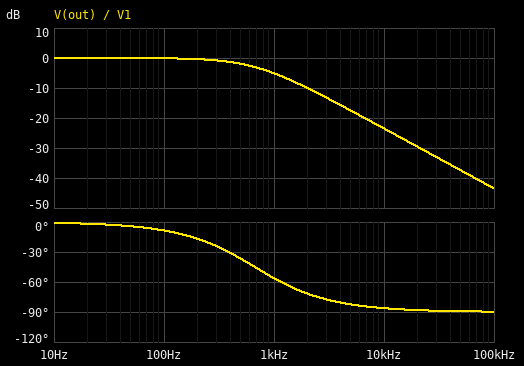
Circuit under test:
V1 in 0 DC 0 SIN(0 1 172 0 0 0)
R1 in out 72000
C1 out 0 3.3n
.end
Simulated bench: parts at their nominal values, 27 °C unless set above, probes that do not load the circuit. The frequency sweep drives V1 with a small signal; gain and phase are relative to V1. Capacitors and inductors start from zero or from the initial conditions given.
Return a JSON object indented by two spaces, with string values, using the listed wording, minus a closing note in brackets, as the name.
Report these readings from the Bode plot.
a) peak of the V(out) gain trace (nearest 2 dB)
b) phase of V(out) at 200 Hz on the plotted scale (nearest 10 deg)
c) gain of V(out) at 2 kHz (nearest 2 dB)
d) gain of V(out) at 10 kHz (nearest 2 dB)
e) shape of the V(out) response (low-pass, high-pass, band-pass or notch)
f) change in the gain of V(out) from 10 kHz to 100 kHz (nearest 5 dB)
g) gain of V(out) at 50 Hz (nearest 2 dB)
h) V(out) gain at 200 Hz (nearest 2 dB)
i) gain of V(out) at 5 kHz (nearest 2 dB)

{
  "peak of the V(out) gain trace": "0 dB",
  "phase of V(out) at 200 Hz on the plotted scale": "-20 deg",
  "gain of V(out) at 2 kHz": "-10 dB",
  "gain of V(out) at 10 kHz": "-24 dB",
  "shape of the V(out) response": "low-pass",
  "change in the gain of V(out) from 10 kHz to 100 kHz": "-20 dB",
  "gain of V(out) at 50 Hz": "0 dB",
  "V(out) gain at 200 Hz": "0 dB",
  "gain of V(out) at 5 kHz": "-18 dB"
}
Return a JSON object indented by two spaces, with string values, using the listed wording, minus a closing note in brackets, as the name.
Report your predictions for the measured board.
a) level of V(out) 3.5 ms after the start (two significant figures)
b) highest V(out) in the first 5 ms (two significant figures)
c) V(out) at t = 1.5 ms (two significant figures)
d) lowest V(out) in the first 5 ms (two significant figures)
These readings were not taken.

{
  "level of V(out) 3.5 ms after the start": "-370 mV",
  "highest V(out) in the first 5 ms": "970 mV",
  "V(out) at t = 1.5 ms": "950 mV",
  "lowest V(out) in the first 5 ms": "-970 mV"
}
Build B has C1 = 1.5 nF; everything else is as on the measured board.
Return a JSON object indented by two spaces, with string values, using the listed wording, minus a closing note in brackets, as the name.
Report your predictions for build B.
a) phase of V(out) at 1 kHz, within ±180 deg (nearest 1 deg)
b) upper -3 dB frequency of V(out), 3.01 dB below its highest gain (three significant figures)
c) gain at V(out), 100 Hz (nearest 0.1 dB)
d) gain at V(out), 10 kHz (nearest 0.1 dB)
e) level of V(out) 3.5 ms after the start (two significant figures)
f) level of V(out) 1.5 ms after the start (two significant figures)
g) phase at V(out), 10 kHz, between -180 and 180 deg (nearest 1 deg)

{
  "phase of V(out) at 1 kHz, within ±180 deg": "-34 deg",
  "upper -3 dB frequency of V(out), 3.01 dB below its highest gain": "1.47 kHz",
  "gain at V(out), 100 Hz": "0 dB",
  "gain at V(out), 10 kHz": "-16.7 dB",
  "level of V(out) 3.5 ms after the start": "-500 mV",
  "level of V(out) 1.5 ms after the start": "990 mV",
  "phase at V(out), 10 kHz, between -180 and 180 deg": "-82 deg"
}
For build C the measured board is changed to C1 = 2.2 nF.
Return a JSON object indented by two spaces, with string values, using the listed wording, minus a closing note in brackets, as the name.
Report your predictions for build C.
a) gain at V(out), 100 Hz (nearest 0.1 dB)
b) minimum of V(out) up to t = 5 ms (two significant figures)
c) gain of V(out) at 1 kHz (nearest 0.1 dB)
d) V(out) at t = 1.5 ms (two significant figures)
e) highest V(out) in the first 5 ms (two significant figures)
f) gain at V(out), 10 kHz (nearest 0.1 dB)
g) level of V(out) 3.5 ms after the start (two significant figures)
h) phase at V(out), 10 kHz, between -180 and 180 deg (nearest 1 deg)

{
  "gain at V(out), 100 Hz": "0 dB",
  "minimum of V(out) up to t = 5 ms": "-990 mV",
  "gain of V(out) at 1 kHz": "-3.0 dB",
  "V(out) at t = 1.5 ms": "980 mV",
  "highest V(out) in the first 5 ms": "990 mV",
  "gain at V(out), 10 kHz": "-20.0 dB",
  "level of V(out) 3.5 ms after the start": "-450 mV",
  "phase at V(out), 10 kHz, between -180 and 180 deg": "-84 deg"
}
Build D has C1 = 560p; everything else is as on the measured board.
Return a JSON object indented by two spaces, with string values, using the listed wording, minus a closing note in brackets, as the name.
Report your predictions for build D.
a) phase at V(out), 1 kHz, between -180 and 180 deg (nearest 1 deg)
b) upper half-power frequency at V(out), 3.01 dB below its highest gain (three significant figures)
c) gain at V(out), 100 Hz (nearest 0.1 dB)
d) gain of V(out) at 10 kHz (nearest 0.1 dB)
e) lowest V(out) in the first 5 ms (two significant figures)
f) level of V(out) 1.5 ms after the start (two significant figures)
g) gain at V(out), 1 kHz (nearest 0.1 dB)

{
  "phase at V(out), 1 kHz, between -180 and 180 deg": "-14 deg",
  "upper half-power frequency at V(out), 3.01 dB below its highest gain": "3.95 kHz",
  "gain at V(out), 100 Hz": "0 dB",
  "gain of V(out) at 10 kHz": "-8.7 dB",
  "lowest V(out) in the first 5 ms": "-1.0 V",
  "level of V(out) 1.5 ms after the start": "1.0 V",
  "gain at V(out), 1 kHz": "-0.3 dB"
}
